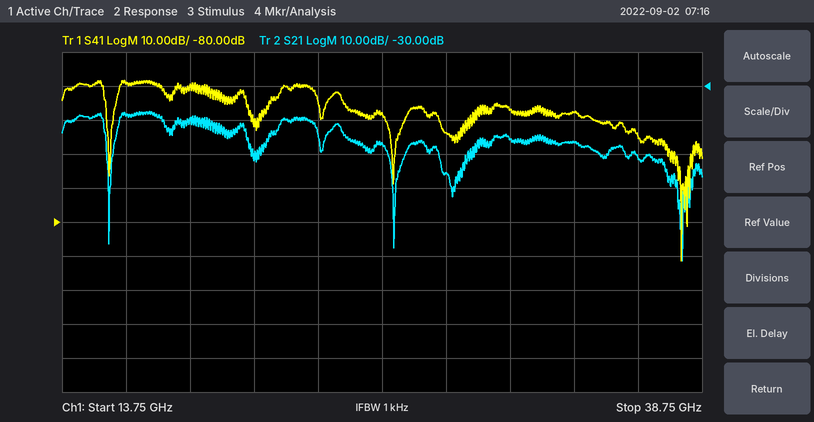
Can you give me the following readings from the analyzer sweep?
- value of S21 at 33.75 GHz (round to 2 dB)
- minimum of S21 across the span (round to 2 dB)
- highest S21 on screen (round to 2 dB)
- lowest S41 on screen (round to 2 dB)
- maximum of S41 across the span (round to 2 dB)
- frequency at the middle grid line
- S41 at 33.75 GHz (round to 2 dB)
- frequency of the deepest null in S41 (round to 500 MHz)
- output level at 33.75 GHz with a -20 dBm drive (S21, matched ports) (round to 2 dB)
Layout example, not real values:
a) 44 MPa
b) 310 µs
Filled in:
a) -46 dB
b) -82 dB
c) -38 dB
d) -92 dB
e) -38 dB
f) 26.25 GHz
g) -48 dB
h) 38.0 GHz
i) -66 dBm
